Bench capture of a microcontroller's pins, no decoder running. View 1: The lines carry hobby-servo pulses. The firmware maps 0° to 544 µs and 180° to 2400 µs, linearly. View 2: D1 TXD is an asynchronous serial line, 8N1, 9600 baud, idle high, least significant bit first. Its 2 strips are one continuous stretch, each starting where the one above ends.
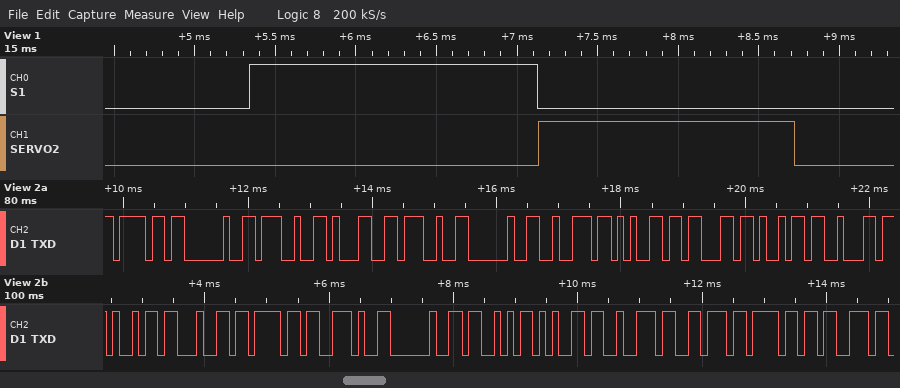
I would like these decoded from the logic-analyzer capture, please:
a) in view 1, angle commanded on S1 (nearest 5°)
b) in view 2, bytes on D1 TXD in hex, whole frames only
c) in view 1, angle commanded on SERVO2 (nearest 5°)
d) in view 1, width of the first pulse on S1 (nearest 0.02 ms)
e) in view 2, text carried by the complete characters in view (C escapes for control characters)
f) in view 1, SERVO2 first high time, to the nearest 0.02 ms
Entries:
120°
0x6F 0x20 0x27 0x31 0x27 0x20 0x72 0x65 0x63 0x69 0x62 0x69 0x64 0x6F 0x2E 0x20 0x53 0x65 0x72 0x76 0x6F 0x73
100°
1.78 ms
"o '1' recibido. Servos"
1.58 ms
